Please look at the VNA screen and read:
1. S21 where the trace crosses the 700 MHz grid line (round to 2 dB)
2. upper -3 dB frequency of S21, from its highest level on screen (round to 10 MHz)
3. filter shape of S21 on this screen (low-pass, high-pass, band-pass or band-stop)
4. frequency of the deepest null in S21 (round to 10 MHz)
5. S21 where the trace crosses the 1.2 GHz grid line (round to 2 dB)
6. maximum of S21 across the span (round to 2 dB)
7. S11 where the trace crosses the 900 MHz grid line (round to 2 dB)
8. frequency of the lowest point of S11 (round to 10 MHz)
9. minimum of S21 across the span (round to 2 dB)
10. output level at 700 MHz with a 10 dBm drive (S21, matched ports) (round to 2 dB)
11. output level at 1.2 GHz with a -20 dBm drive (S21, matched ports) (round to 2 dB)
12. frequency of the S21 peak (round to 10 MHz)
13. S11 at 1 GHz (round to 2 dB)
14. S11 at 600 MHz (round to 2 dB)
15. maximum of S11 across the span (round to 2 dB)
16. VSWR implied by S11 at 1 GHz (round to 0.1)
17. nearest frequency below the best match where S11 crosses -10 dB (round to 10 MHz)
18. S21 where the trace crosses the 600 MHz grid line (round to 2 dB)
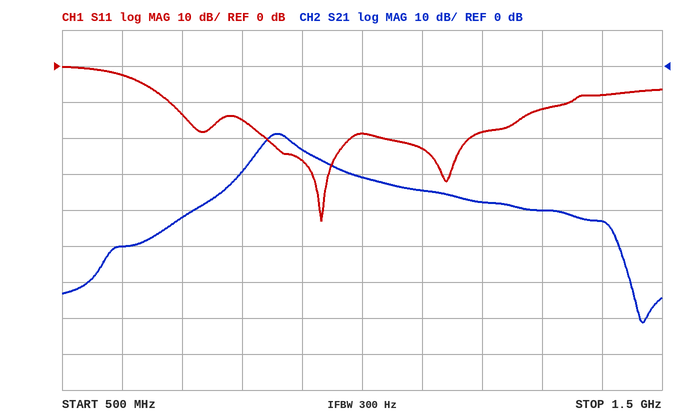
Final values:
-42 dB
890 MHz
band-pass
1.47 GHz
-38 dB
-18 dB
-26 dB
930 MHz
-72 dB
-32 dBm
-58 dBm
860 MHz
-18 dB
-2 dB
0 dB
1.3
680 MHz
-50 dB
